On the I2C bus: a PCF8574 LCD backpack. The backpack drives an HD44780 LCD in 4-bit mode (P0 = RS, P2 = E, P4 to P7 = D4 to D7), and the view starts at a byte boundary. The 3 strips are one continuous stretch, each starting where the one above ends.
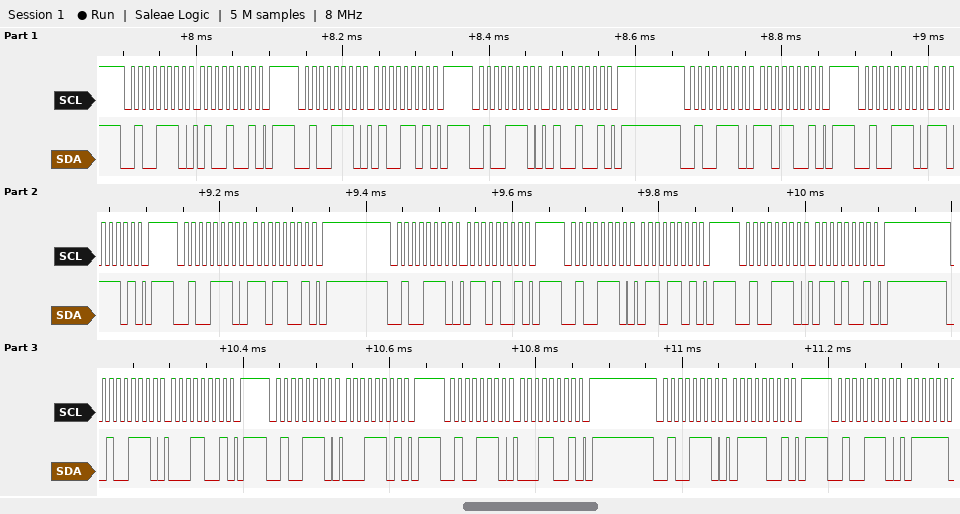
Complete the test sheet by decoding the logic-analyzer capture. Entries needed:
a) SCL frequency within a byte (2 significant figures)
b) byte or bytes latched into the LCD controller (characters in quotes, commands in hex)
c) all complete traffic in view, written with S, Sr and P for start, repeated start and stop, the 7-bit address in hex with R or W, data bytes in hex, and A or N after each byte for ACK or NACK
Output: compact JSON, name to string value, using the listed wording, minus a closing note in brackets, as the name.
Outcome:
{"SCL frequency within a byte": "100 kHz", "byte or bytes latched into the LCD controller": "'M' 'a'", "all complete traffic in view, written with S, Sr and P for start, repeated start and stop, the 7-bit address in hex with R or W, data bytes in hex, and A or N after each byte for ACK or NACK": "S 27W A 49 A P S 27W A 4D A P S 27W A 49 A P S 27W A D9 A P S 27W A DD A P S 27W A D9 A P S 27W A 69 A P S 27W A 6D A P S 27W A 69 A P S 27W A 19 A P S 27W A 1D A P S 27W A 19 A P S 27W A 79 A P S 27W A"}
